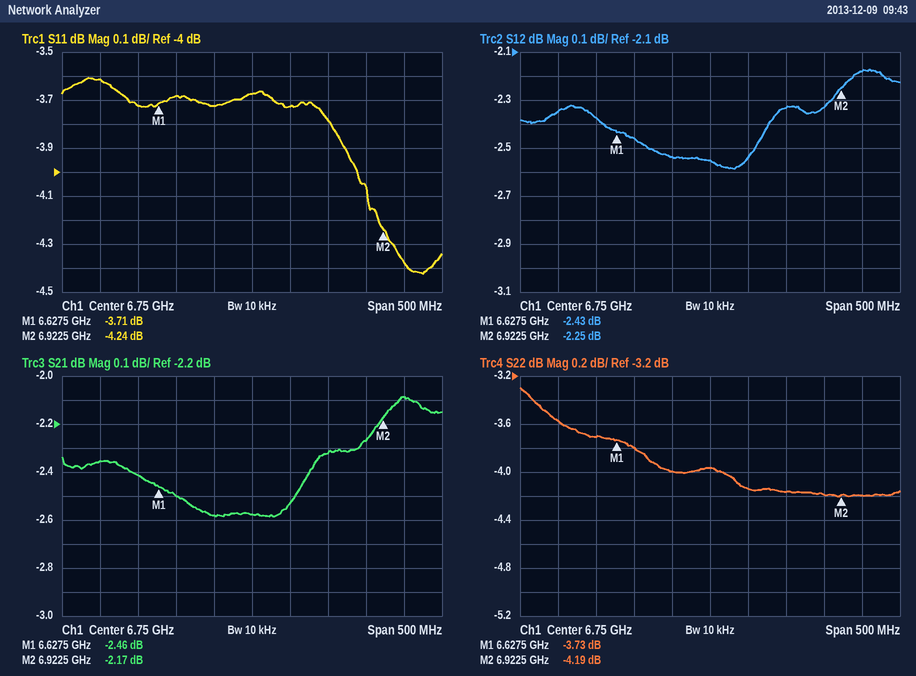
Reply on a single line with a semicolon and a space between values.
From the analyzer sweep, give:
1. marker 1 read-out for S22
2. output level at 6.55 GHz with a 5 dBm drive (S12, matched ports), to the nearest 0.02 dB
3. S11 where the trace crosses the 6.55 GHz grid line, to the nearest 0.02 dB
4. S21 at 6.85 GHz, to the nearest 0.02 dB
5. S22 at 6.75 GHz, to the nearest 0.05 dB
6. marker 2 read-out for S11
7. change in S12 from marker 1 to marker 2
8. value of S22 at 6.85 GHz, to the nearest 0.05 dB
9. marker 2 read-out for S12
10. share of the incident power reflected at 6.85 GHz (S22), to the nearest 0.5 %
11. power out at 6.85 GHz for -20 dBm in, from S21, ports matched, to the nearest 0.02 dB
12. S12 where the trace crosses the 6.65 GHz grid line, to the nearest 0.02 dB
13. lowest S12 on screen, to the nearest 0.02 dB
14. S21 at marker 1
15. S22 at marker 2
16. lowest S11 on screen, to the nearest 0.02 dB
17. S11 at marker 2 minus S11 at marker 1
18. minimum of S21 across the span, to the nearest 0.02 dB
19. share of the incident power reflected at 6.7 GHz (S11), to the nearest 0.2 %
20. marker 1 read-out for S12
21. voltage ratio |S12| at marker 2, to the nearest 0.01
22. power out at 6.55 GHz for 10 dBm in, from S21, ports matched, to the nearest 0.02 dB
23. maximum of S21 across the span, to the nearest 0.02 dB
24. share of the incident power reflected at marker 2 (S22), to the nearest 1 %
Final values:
-3.73 dB; 2.66 dBm; -3.62 dB; -2.32 dB; -3.95 dB; -4.24 dB; 0.18 dB; -4.15 dB; -2.25 dB; 38.5 %; -22.32 dBm; -2.46 dB; -2.58 dB; -2.46 dB; -4.19 dB; -4.42 dB; -0.53 dB; -2.58 dB; 42.4 %; -2.43 dB; 0.77; 7.64 dBm; -2.08 dB; 38 %
